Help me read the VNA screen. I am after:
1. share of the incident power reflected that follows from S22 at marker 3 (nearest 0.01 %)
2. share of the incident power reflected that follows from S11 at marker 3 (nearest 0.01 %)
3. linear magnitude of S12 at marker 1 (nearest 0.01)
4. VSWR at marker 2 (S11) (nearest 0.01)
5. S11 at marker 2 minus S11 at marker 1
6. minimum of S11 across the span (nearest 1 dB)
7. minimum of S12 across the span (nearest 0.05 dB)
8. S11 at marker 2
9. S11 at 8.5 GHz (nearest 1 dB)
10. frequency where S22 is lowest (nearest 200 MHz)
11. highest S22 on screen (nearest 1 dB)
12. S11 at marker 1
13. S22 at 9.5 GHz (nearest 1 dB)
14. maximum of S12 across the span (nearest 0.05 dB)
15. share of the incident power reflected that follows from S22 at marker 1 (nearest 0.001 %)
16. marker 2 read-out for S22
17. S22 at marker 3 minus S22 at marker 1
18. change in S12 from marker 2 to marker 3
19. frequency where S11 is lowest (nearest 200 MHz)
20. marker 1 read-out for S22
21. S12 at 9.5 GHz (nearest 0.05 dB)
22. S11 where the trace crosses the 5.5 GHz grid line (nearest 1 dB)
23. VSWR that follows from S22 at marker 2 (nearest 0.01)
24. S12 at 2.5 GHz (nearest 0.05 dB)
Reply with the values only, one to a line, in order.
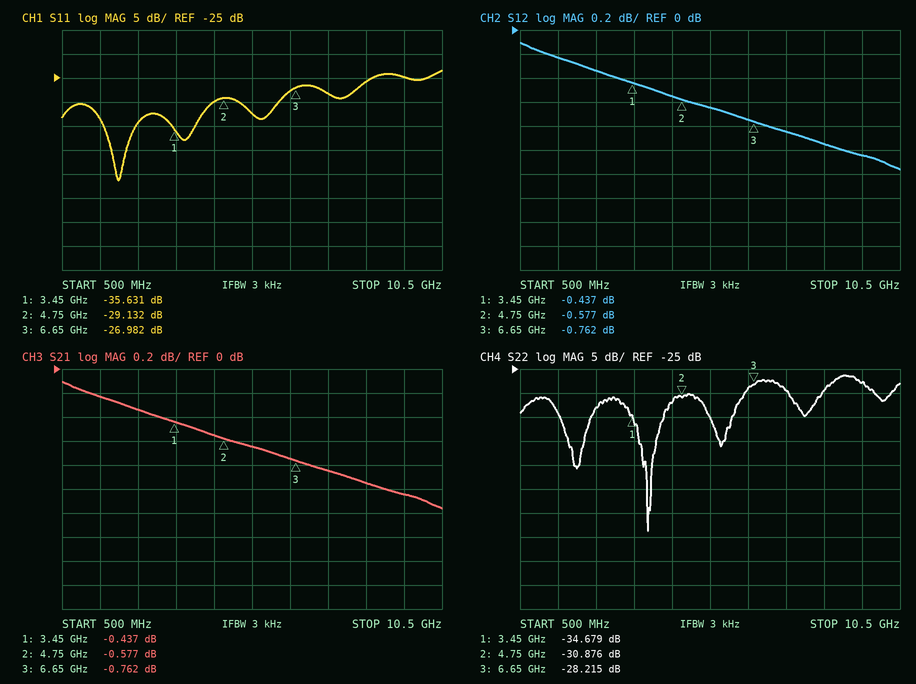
0.15 %
0.20 %
0.95
1.07
6.499 dB
-46 dB
-1.15 dB
-29.132 dB
-26 dB
3.8 GHz
-26 dB
-35.631 dB
-28 dB
-0.10 dB
0.034 %
-30.876 dB
6.464 dB
-0.185 dB
2.0 GHz
-34.679 dB
-1.05 dB
-32 dB
1.06
-0.35 dB
